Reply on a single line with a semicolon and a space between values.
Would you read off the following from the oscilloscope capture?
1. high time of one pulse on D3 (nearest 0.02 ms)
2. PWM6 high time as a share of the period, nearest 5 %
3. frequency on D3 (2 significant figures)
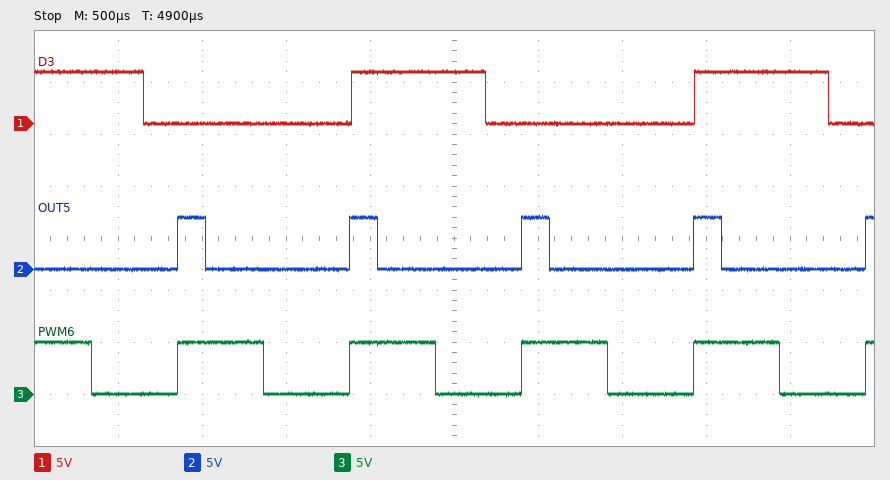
0.80 ms; 50 %; 490 Hz
